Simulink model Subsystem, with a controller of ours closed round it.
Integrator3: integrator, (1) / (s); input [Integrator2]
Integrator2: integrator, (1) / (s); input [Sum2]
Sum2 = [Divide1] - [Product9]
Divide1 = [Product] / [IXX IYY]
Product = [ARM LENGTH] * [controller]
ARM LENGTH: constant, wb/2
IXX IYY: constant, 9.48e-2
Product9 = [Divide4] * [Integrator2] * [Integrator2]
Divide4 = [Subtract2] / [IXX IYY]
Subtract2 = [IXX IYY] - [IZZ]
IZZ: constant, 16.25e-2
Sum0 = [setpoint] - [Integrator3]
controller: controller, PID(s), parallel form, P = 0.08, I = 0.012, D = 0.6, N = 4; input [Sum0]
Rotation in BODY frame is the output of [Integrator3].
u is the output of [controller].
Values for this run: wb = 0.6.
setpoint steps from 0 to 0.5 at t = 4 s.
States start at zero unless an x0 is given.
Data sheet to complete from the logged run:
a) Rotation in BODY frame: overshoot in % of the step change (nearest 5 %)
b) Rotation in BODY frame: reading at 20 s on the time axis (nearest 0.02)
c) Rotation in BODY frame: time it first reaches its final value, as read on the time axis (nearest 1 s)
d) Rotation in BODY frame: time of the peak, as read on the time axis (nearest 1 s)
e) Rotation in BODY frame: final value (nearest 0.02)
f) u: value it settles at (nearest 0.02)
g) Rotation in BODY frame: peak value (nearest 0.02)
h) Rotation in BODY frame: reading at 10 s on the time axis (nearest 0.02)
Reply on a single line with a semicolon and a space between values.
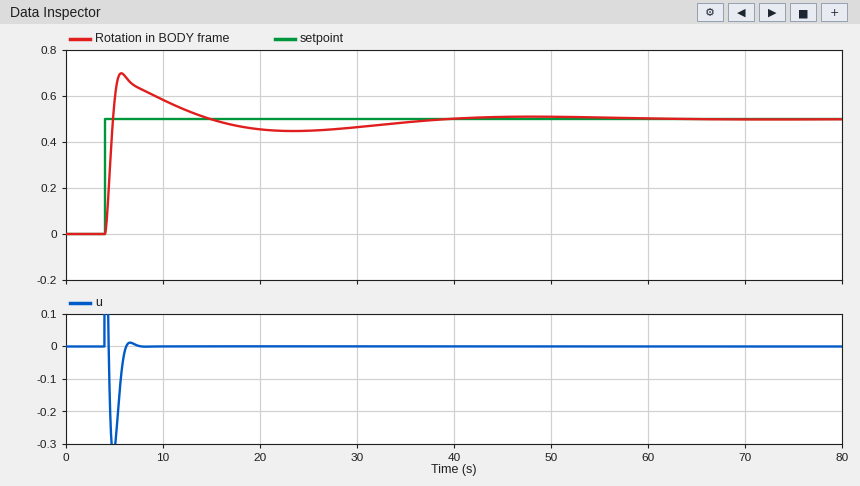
40 %; 0.46; 5 s; 6 s; 0.50; 0.00; 0.70; 0.58
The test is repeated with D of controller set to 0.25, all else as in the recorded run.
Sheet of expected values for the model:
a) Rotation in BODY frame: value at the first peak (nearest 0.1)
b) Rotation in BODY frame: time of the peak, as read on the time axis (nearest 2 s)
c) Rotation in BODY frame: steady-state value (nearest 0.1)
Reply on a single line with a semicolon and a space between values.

0.8; 8 s; 0.5
